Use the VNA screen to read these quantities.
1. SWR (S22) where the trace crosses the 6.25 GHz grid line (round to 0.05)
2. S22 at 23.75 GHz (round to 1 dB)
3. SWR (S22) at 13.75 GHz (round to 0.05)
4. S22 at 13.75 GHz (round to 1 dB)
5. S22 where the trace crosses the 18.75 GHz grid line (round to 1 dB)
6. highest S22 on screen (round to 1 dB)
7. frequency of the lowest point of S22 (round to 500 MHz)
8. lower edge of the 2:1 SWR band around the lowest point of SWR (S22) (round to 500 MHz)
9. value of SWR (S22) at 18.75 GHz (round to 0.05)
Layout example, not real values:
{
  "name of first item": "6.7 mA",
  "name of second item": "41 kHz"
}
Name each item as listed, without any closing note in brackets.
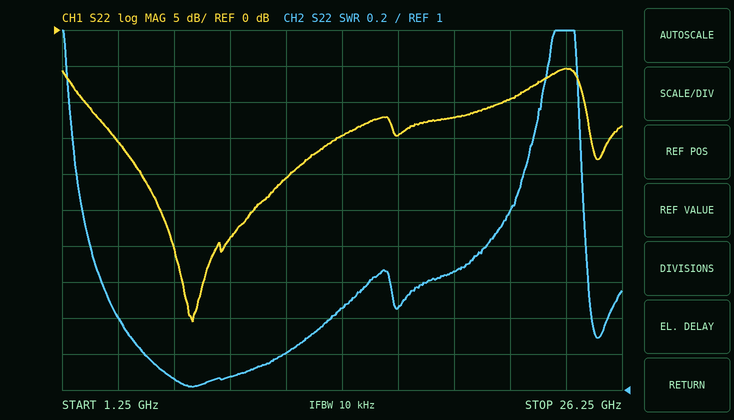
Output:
{
  "SWR (S22) where the trace crosses the 6.25 GHz grid line": "1.05",
  "S22 at 23.75 GHz": "-5 dB",
  "SWR (S22) at 13.75 GHz": "1.45",
  "S22 at 13.75 GHz": "-15 dB",
  "S22 where the trace crosses the 18.75 GHz grid line": "-12 dB",
  "highest S22 on screen": "-5 dB",
  "frequency of the lowest point of S22": "7.0 GHz",
  "lower edge of the 2:1 SWR band around the lowest point of SWR (S22)": "2.0 GHz",
  "value of SWR (S22) at 18.75 GHz": "1.65"
}
